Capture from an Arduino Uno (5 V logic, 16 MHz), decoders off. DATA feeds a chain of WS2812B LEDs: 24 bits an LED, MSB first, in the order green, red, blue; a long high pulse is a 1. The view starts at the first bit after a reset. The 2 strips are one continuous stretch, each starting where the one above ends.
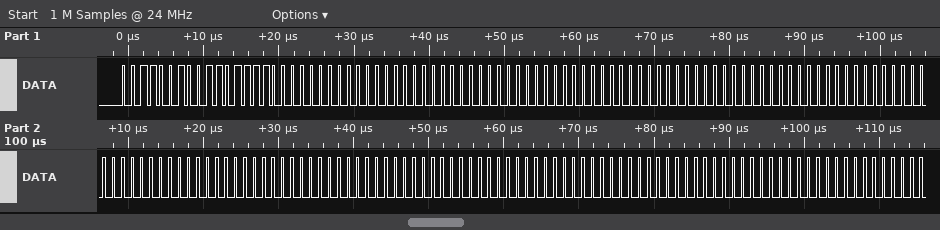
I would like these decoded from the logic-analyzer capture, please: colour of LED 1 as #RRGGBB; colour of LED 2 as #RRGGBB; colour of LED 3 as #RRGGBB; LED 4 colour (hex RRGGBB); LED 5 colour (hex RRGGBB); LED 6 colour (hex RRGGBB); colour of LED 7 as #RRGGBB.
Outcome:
#6F3200
#000000
#000000
#000000
#000000
#000000
#000000
